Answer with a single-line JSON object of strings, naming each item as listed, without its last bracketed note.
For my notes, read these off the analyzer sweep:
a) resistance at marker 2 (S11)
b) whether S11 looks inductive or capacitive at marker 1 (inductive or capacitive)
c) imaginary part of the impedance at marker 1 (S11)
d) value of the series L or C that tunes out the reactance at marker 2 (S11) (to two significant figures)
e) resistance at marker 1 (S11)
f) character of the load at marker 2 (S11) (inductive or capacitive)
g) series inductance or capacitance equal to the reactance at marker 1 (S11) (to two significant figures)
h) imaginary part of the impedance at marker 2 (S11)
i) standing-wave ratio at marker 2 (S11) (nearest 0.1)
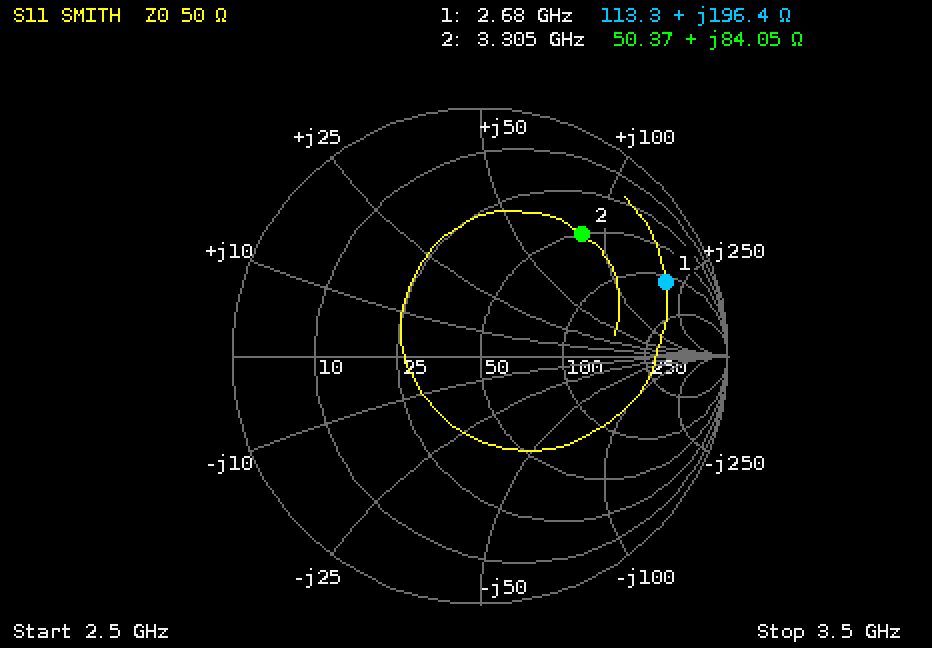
{"resistance at marker 2": "50.37 Ω", "whether S11 looks inductive or capacitive at marker 1": "inductive", "imaginary part of the impedance at marker 1": "+196.4 Ω", "value of the series L or C that tunes out the reactance at marker 2 (S11)": "570 fF", "resistance at marker 1": "113.3 Ω", "character of the load at marker 2 (S11)": "inductive", "series inductance or capacitance equal to the reactance at marker 1 (S11)": "12 nH", "imaginary part of the impedance at marker 2": "+84.05 Ω", "standing-wave ratio at marker 2 (S11)": "4.6"}
